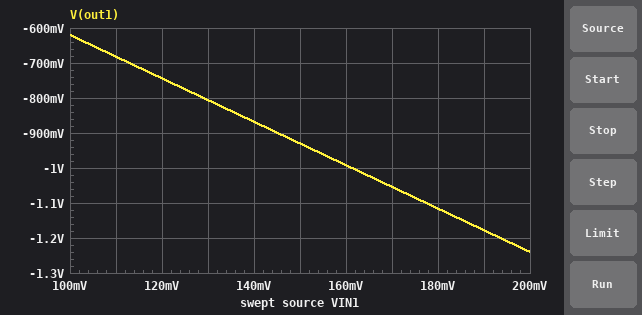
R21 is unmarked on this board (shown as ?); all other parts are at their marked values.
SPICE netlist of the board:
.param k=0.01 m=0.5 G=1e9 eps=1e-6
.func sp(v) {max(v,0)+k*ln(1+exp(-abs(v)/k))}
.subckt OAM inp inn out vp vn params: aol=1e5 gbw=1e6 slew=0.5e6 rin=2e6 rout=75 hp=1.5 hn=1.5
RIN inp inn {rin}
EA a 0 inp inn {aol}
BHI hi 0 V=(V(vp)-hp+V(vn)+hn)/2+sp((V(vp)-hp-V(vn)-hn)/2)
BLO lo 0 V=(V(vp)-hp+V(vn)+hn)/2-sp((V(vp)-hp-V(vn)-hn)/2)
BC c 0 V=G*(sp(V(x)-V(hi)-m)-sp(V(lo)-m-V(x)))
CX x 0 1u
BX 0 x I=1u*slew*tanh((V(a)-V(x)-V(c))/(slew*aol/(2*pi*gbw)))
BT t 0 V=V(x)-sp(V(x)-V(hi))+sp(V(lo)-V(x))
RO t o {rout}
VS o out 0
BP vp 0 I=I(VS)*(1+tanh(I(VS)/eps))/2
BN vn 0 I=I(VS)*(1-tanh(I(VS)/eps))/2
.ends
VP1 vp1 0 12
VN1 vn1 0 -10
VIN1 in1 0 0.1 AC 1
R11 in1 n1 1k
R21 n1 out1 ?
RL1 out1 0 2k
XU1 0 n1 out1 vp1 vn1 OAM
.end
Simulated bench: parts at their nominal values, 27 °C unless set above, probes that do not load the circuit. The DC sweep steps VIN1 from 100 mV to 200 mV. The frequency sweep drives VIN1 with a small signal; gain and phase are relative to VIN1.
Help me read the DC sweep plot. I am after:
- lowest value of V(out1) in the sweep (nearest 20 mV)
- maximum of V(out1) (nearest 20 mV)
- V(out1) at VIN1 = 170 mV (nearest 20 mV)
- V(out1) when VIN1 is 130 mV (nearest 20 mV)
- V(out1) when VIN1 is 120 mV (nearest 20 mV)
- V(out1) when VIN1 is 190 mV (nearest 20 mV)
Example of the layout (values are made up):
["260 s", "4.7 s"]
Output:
["-1.24 V", "-620 mV", "-1.06 V", "-800 mV", "-740 mV", "-1.18 V"]
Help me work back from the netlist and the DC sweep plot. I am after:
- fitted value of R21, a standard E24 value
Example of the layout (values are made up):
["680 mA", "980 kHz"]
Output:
["6.2 kΩ"]
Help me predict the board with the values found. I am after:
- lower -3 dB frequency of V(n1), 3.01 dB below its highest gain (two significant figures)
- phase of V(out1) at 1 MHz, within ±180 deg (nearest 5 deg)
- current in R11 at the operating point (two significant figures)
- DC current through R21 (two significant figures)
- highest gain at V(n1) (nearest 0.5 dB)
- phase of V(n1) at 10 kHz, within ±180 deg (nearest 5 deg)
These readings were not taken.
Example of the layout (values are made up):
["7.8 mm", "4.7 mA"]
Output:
["130 kHz", "95 deg", "100 µA", "100 µA", "-1.5 dB", "85 deg"]
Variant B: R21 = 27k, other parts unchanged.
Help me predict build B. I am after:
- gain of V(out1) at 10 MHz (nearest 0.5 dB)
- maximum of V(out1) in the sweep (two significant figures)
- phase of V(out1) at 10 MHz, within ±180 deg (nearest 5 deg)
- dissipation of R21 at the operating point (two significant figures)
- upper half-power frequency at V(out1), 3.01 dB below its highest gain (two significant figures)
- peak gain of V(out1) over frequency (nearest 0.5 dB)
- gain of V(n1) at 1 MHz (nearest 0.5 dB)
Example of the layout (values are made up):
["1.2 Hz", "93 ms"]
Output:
["-20.5 dB", "-2.7 V", "90 deg", "270 µW", "34 kHz", "28.5 dB", "-0.5 dB"]
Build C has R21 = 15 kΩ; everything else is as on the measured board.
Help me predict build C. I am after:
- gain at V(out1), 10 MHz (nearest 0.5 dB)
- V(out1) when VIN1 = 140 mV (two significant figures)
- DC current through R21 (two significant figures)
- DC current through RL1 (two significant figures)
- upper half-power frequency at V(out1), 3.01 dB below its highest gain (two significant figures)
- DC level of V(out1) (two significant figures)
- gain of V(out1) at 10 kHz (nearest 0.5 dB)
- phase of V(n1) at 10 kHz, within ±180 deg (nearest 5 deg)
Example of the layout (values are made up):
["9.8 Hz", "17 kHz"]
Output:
["-21.0 dB", "-2.1 V", "100 µA", "750 µA", "60 kHz", "-1.5 V", "23.5 dB", "80 deg"]
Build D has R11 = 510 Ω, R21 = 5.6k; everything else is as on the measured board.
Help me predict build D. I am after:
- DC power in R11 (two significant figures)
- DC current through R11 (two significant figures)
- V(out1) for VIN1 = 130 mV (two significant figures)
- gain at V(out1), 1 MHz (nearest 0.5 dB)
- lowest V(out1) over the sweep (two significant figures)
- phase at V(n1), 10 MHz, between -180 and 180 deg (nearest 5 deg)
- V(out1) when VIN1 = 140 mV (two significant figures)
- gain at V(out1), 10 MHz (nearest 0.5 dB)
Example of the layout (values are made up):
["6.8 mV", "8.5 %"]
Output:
["20 µW", "200 µA", "-1.4 V", "-1.0 dB", "-2.2 V", "0 deg", "-1.5 V", "-21.0 dB"]
